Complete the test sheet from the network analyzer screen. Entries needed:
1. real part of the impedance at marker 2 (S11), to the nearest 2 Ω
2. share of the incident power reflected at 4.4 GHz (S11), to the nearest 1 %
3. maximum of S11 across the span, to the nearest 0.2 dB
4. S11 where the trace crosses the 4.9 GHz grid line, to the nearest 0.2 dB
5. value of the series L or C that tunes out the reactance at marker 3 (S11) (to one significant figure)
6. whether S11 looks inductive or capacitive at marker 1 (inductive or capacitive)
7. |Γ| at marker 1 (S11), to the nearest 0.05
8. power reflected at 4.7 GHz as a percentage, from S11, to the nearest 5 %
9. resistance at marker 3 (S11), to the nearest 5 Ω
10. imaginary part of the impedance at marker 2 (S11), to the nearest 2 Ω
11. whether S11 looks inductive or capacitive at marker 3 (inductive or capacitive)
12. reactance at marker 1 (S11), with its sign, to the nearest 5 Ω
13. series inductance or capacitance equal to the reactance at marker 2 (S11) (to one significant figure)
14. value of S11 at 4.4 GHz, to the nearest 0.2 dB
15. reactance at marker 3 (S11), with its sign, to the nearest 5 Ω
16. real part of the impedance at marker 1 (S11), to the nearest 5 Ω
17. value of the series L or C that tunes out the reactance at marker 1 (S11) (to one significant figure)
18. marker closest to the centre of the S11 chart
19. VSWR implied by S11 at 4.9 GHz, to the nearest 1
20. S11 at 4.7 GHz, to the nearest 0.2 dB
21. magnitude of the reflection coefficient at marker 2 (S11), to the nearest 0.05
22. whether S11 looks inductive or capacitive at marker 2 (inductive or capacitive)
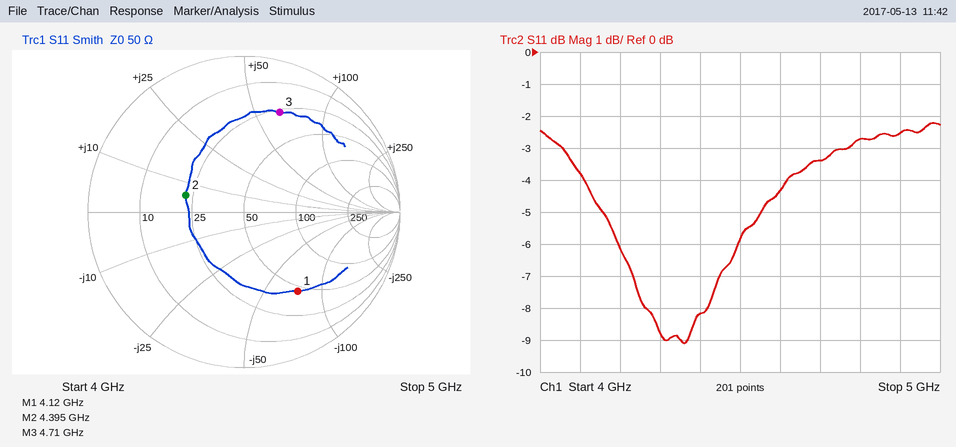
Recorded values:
22 Ω
15 %
-2.2 dB
-2.6 dB
500 fF
capacitive
0.60
45 %
25 Ω
+6 Ω
inductive
-75 Ω
200 pH
-8.2 dB
+65 Ω
45 Ω
3 nH
marker 2
7
-3.4 dB
0.40
inductive
